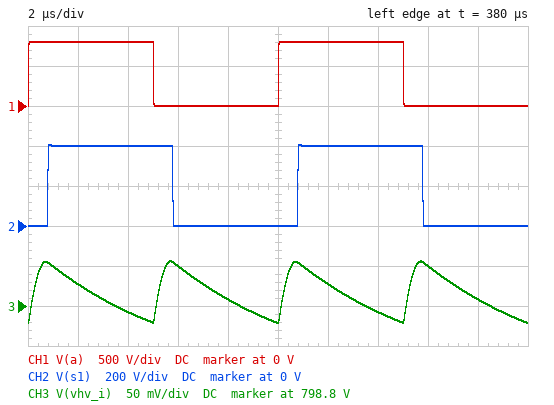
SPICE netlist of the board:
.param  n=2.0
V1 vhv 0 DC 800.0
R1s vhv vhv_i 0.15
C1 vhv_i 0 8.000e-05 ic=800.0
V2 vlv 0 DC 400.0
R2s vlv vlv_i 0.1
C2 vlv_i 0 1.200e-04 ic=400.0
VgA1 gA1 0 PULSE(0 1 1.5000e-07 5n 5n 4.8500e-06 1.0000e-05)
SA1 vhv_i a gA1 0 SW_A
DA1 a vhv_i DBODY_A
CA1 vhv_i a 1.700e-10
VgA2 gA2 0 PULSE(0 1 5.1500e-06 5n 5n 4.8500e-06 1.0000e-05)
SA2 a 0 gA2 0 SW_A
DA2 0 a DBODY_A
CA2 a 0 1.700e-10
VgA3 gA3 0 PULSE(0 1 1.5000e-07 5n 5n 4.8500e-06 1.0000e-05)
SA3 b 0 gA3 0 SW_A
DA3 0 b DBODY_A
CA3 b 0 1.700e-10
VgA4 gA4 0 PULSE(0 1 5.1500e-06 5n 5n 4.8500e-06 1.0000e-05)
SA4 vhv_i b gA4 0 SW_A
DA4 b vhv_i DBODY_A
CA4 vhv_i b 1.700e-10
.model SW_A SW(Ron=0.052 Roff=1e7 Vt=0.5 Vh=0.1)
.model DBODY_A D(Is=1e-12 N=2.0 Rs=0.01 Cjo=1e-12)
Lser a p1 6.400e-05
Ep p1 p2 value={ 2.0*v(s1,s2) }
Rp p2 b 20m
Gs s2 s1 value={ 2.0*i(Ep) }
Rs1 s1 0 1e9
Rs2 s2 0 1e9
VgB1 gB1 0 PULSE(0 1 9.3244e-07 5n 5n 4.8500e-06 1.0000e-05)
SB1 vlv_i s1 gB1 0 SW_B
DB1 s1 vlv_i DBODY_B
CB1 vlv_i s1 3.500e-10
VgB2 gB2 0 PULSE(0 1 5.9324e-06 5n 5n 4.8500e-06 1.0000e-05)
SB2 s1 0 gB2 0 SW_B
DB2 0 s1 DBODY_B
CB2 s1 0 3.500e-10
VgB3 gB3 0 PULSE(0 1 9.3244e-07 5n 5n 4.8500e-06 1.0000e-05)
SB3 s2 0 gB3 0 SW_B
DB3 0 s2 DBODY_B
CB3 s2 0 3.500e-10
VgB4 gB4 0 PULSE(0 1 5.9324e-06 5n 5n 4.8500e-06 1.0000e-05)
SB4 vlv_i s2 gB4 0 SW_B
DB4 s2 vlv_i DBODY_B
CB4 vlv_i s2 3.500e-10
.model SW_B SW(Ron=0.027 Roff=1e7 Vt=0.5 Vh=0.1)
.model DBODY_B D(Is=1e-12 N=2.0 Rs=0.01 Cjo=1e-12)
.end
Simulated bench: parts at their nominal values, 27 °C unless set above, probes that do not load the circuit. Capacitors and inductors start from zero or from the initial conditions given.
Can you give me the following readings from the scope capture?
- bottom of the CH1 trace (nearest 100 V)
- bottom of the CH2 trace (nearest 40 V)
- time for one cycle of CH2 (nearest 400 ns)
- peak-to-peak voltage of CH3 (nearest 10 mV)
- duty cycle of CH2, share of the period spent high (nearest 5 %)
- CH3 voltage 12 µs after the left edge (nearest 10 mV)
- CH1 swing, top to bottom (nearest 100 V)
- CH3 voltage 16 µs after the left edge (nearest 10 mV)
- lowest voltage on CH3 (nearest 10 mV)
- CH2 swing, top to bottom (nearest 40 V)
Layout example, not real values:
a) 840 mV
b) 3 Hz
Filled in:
a) 0 V
b) 0 V
c) 10.0 µs
d) 80 mV
e) 50 %
f) 798.78 V
g) 800 V
h) 798.80 V
i) 798.73 V
j) 400 V
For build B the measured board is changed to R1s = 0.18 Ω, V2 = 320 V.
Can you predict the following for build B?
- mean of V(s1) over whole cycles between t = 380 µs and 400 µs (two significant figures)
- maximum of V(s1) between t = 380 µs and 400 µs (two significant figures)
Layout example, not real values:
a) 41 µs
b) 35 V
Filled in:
a) 160 V
b) 320 V
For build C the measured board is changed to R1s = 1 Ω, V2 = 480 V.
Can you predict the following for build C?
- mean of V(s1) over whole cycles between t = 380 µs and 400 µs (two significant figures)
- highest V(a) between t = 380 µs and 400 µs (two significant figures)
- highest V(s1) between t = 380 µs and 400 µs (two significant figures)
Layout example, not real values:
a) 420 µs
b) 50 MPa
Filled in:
a) 240 V
b) 790 V
c) 480 V
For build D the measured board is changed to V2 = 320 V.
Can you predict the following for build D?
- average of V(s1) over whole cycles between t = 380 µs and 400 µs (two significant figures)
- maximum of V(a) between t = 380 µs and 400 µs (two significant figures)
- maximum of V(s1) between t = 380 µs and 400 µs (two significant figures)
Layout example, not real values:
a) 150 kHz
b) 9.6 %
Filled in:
a) 160 V
b) 800 V
c) 320 V
